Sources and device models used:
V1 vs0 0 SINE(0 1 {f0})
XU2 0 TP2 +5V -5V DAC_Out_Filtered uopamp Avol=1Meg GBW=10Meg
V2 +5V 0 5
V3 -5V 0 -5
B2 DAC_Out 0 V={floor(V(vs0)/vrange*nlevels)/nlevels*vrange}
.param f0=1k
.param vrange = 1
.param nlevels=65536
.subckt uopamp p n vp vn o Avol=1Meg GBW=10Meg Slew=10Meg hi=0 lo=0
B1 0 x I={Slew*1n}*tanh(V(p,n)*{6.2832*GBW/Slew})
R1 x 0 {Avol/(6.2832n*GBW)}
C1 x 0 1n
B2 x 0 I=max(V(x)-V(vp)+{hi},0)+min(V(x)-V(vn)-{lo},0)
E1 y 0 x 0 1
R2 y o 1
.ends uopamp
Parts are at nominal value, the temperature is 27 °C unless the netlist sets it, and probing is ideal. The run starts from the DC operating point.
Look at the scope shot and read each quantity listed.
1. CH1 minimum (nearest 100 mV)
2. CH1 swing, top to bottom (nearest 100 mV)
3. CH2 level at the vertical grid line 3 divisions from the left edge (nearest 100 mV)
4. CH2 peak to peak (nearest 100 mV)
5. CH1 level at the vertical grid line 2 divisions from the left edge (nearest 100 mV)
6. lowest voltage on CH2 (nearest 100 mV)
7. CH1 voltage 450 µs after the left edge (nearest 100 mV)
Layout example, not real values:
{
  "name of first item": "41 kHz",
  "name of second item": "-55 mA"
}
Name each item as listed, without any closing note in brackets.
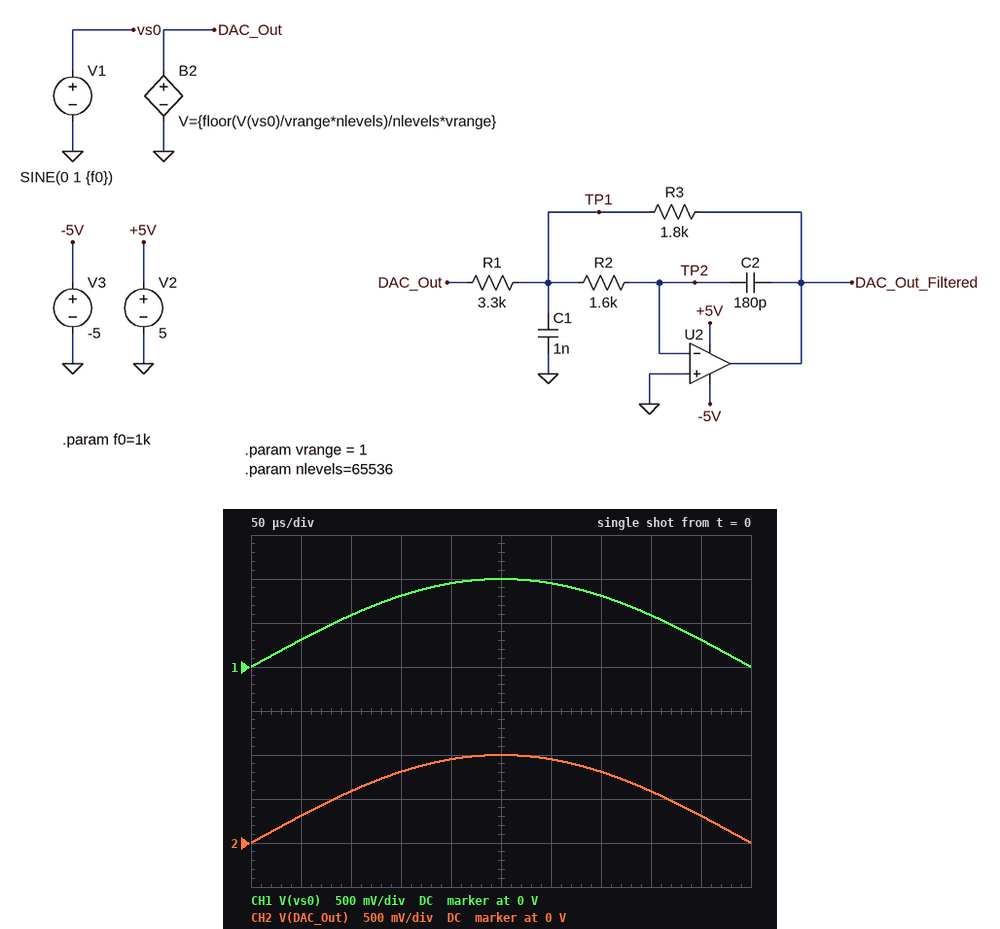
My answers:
{
  "CH1 minimum": "0 V",
  "CH1 swing, top to bottom": "1.0 V",
  "CH2 level at the vertical grid line 3 divisions from the left edge": "800 mV",
  "CH2 peak to peak": "1.0 V",
  "CH1 level at the vertical grid line 2 divisions from the left edge": "600 mV",
  "lowest voltage on CH2": "0 V",
  "CH1 voltage 450 µs after the left edge": "300 mV"
}
